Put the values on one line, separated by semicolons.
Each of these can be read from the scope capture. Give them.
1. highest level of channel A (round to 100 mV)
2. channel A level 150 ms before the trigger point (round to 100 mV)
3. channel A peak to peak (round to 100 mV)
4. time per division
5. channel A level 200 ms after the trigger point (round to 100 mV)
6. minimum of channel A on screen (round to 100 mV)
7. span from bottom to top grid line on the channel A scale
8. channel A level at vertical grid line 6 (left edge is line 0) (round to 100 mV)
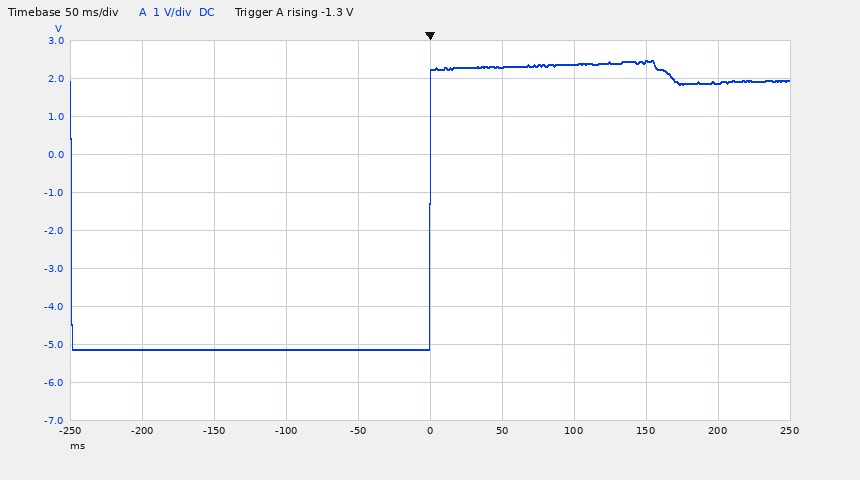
2.5 V; -5.1 V; 7.6 V; 50 ms; 1.9 V; -5.1 V; 10 V; 2.3 V
